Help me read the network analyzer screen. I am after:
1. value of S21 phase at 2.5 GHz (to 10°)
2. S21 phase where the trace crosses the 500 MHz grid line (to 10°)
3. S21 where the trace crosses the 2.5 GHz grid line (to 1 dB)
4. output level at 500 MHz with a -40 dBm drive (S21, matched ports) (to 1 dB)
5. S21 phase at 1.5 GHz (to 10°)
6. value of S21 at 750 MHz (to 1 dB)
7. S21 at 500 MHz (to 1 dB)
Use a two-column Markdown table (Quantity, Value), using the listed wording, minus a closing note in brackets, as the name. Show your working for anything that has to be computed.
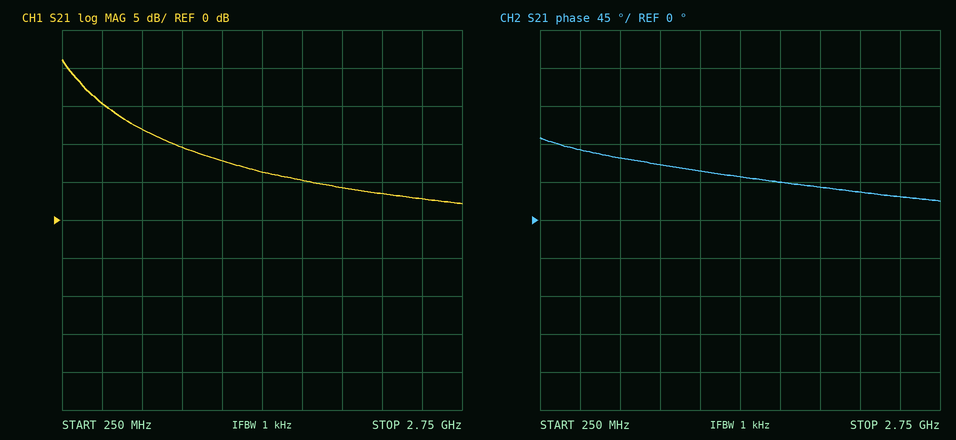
| Quantity | Value |
|---|---|
| value of S21 phase at 2.5 GHz | 30° |
| S21 phase where the trace crosses the 500 MHz grid line | 80° |
| S21 where the trace crosses the 2.5 GHz grid line | 3 dB |
| output level at 500 MHz with a -40 dBm drive (S21, matched ports) | -40 dBm + (15 dB) = -25 dBm |
| S21 phase at 1.5 GHz | 50° |
| value of S21 at 750 MHz | 12 dB |
| S21 at 500 MHz | 15 dB |
